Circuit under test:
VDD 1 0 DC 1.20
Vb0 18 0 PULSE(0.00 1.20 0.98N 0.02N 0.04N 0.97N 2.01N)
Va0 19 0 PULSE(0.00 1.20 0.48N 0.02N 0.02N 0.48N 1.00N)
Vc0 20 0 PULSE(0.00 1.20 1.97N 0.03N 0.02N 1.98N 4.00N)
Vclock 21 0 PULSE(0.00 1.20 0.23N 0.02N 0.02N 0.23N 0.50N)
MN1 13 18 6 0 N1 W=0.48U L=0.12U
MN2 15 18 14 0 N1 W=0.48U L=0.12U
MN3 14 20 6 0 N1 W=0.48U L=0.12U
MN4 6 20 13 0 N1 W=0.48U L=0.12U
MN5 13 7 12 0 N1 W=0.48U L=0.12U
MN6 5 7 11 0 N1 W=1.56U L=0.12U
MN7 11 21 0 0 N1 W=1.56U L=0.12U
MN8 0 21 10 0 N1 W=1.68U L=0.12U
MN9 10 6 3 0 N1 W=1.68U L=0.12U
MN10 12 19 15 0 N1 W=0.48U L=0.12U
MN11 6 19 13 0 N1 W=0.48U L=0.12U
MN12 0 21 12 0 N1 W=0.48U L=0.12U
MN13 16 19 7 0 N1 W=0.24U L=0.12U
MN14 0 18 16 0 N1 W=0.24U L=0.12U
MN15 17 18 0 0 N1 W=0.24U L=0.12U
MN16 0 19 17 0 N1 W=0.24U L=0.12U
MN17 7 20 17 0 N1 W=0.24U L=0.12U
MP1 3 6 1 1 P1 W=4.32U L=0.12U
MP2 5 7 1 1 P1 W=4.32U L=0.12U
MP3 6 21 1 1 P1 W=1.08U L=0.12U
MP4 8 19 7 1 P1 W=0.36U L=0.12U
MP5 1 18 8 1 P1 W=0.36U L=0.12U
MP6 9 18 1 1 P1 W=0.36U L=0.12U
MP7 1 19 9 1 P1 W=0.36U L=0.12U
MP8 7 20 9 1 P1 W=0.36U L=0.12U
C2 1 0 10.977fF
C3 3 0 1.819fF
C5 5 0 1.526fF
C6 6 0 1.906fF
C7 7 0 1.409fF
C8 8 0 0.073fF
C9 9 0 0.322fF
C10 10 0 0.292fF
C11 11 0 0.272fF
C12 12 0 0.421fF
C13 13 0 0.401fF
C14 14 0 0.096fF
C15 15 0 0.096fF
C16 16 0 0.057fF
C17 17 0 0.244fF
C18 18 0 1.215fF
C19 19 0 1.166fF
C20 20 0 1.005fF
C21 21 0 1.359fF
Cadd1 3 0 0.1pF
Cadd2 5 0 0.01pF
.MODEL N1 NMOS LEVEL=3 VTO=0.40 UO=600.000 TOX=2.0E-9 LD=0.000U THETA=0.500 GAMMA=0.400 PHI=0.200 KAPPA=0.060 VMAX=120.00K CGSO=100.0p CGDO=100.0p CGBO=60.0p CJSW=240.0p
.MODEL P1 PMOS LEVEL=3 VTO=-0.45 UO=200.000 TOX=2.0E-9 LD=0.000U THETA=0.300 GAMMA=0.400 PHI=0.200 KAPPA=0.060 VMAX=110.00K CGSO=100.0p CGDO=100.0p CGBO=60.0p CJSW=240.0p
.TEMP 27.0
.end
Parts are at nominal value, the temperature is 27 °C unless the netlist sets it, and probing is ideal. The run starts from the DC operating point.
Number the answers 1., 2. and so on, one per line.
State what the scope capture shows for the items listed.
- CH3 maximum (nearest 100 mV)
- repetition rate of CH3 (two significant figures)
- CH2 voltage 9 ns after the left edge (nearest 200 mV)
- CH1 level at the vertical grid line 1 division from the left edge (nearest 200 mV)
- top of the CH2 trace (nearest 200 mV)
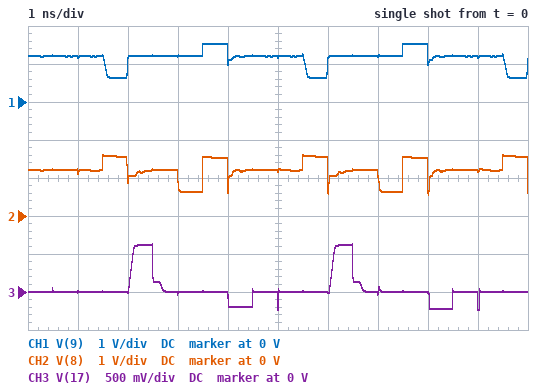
1. 600 mV
2. 250 MHz
3. 1.2 V
4. 1.2 V
5. 1.6 V
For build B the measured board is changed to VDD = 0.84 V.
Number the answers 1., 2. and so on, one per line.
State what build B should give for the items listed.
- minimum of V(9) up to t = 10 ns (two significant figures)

1. 550 mV
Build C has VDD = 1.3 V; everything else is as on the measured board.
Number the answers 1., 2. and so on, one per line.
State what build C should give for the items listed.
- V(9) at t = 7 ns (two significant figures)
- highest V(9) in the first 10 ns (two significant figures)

1. 1.3 V
2. 1.6 V
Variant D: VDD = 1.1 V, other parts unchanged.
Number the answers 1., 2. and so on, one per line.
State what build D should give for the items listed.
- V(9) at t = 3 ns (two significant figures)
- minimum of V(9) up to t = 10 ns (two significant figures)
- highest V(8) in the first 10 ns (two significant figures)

1. 1.1 V
2. 610 mV
3. 1.6 V
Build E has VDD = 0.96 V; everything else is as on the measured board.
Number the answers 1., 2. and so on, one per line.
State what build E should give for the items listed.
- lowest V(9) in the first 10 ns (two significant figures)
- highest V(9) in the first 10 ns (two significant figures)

1. 580 mV
2. 1.4 V
